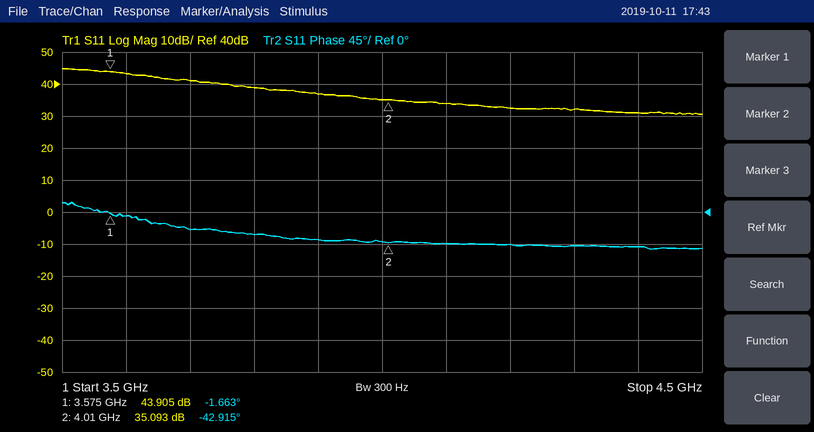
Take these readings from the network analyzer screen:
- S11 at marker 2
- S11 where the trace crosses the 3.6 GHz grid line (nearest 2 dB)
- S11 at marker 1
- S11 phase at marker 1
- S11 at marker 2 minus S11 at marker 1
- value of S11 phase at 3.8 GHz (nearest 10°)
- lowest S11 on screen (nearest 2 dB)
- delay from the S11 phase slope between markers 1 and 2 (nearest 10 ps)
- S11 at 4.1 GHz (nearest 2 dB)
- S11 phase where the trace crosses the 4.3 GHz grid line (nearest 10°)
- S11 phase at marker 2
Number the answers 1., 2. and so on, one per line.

1. 35.093 dB
2. 44 dB
3. 43.905 dB
4. -1.663°
5. -8.812 dB
6. -30°
7. 30 dB
8. 260 ps
9. 34 dB
10. -50°
11. -42.915°
